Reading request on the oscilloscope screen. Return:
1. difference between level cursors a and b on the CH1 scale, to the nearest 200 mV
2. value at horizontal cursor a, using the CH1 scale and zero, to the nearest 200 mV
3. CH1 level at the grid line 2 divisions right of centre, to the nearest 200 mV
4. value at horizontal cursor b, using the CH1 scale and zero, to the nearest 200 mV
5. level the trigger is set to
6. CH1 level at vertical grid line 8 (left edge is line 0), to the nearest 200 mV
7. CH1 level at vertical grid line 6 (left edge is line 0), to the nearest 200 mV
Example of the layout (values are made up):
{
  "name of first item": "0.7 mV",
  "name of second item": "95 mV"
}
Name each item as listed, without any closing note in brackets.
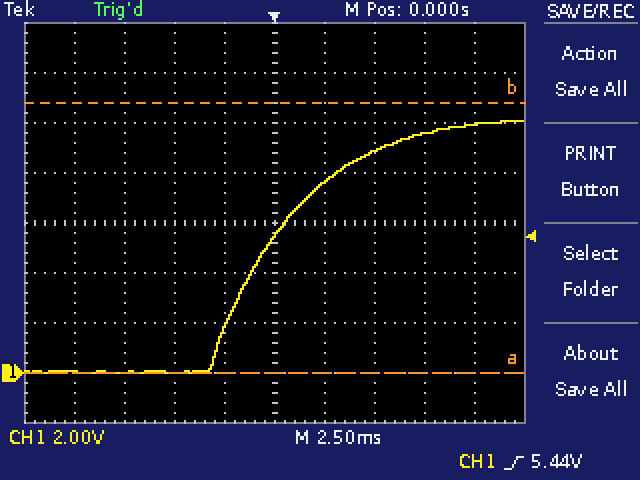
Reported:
{
  "difference between level cursors a and b on the CH1 scale, to the nearest 200 mV": "10.8 V",
  "value at horizontal cursor a, using the CH1 scale and zero, to the nearest 200 mV": "0.0 V",
  "CH1 level at the grid line 2 divisions right of centre, to the nearest 200 mV": "8.8 V",
  "value at horizontal cursor b, using the CH1 scale and zero, to the nearest 200 mV": "10.8 V",
  "level the trigger is set to": "5.44 V",
  "CH1 level at vertical grid line 8 (left edge is line 0), to the nearest 200 mV": "9.6 V",
  "CH1 level at vertical grid line 6 (left edge is line 0), to the nearest 200 mV": "7.6 V"
}
